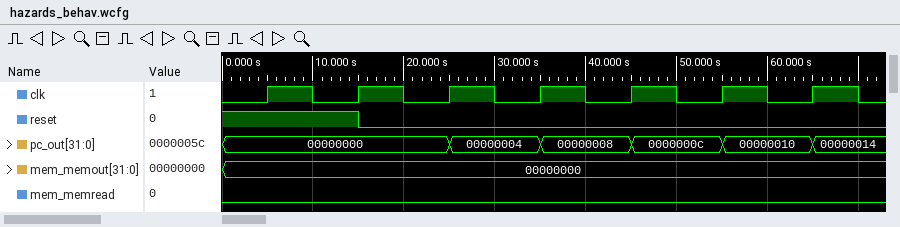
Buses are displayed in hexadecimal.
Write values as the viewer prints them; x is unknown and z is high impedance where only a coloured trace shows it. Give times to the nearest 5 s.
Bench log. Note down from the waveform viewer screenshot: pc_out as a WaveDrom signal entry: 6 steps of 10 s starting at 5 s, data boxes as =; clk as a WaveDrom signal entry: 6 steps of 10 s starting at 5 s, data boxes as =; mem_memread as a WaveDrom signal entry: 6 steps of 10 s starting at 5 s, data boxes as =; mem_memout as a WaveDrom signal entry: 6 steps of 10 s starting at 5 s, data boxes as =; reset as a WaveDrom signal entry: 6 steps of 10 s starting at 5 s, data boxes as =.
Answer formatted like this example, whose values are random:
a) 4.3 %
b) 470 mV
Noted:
a) {name: 'pc_out', wave: '=.====', data: '00000000 00000004 00000008 0000000c 00000010'}
b) {name: 'clk', wave: 'p.....'}
c) {name: 'mem_memread', wave: '0.....'}
d) {name: 'mem_memout', wave: '=.....', data: '00000000'}
e) {name: 'reset', wave: '10....'}
